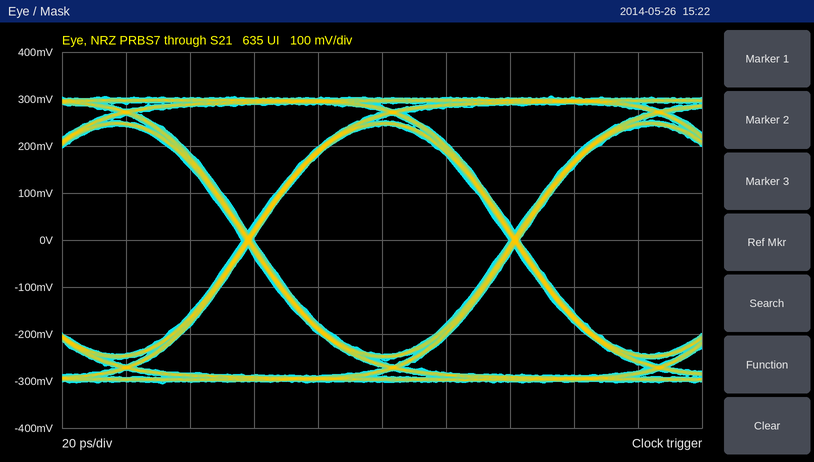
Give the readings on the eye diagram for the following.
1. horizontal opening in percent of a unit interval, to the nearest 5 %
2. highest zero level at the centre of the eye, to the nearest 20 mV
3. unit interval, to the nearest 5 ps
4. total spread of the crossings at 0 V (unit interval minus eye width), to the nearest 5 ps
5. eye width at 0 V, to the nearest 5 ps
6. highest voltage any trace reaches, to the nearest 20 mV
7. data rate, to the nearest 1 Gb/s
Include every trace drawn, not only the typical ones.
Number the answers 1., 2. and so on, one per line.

1. 95 %
2. -240 mV
3. 85 ps
4. 5 ps
5. 80 ps
6. 300 mV
7. 12 Gb/s
